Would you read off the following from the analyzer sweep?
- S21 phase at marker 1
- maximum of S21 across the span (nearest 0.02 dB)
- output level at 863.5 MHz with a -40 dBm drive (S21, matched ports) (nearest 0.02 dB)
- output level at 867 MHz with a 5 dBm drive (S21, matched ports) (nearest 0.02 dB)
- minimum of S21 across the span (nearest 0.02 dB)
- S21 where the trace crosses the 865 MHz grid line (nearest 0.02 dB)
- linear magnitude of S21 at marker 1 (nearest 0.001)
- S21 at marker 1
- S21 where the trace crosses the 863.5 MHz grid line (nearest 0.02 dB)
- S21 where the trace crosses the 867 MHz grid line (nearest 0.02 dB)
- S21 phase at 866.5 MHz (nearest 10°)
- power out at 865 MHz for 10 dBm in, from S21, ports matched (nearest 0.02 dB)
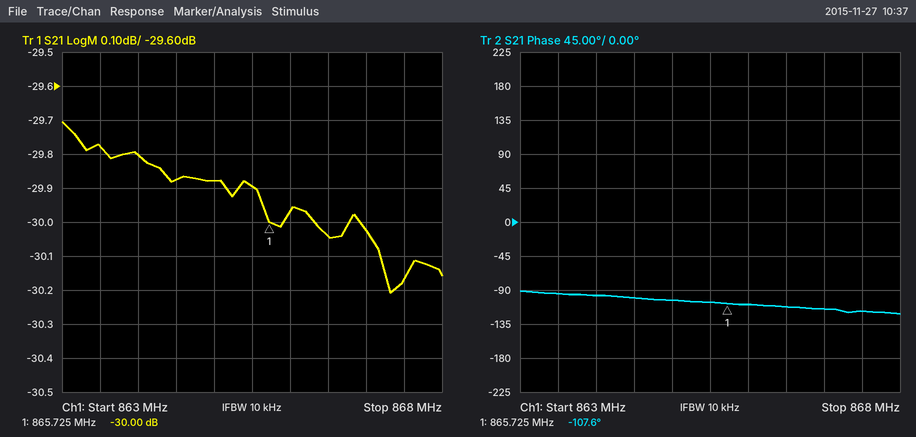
-107.6°
-29.70 dB
-69.78 dBm
-25.02 dBm
-30.20 dB
-29.88 dB
0.032
-30.00 dB
-29.78 dB
-30.02 dB
-110°
-19.88 dBm
